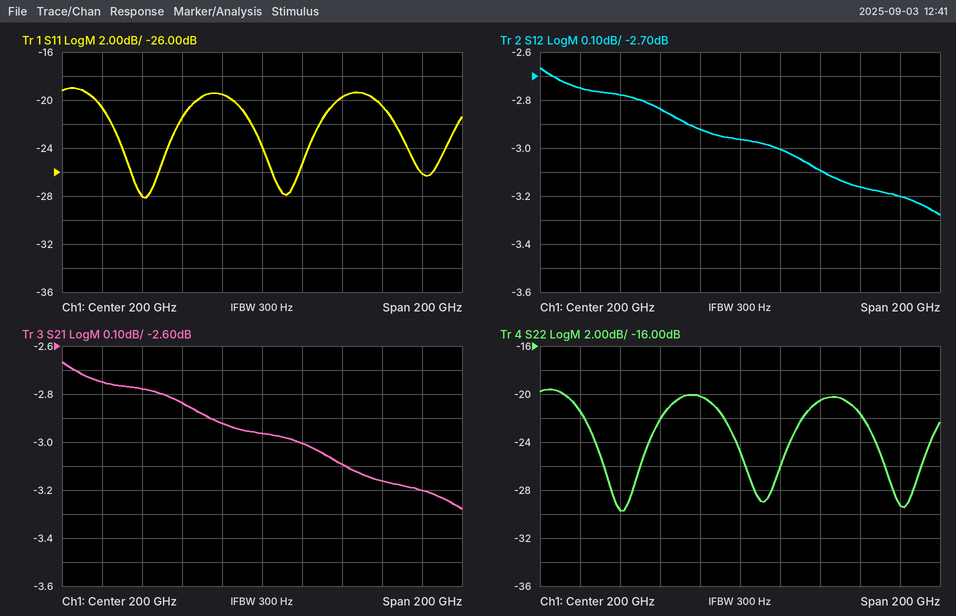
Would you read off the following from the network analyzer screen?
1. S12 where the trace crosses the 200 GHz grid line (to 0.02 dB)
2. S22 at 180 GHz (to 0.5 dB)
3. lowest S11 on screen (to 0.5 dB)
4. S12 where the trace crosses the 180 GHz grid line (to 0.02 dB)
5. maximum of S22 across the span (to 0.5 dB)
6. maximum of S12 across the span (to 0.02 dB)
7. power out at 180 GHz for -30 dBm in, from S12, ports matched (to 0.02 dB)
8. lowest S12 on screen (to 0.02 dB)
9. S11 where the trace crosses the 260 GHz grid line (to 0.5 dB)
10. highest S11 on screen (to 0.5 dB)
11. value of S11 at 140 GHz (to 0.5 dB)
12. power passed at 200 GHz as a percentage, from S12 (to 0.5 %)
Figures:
-2.96 dB
-20.0 dB
-28.0 dB
-2.92 dB
-19.5 dB
-2.66 dB
-32.92 dBm
-3.28 dB
-20.5 dB
-19.0 dB
-28.0 dB
50.5 %
